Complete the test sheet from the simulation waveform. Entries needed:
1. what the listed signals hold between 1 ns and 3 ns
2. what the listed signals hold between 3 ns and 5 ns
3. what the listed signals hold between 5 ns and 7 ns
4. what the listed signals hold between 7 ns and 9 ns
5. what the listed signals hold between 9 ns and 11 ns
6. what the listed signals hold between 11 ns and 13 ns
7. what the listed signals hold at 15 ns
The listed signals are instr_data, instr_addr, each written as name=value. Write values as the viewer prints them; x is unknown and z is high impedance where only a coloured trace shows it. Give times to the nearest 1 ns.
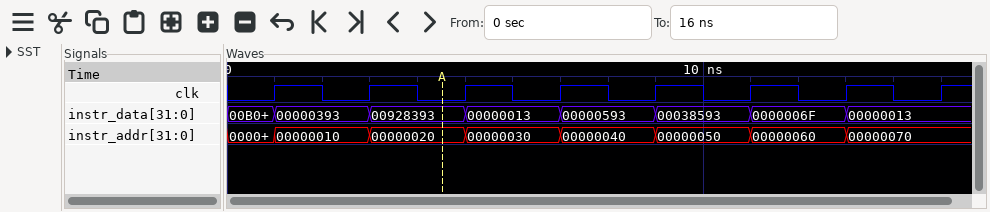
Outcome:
instr_data=00000393, instr_addr=00000010
instr_data=00928393, instr_addr=00000020
instr_data=00000013, instr_addr=00000030
instr_data=00000593, instr_addr=00000040
instr_data=00038593, instr_addr=00000050
instr_data=0000006F, instr_addr=00000060
instr_data=00000013, instr_addr=00000070
